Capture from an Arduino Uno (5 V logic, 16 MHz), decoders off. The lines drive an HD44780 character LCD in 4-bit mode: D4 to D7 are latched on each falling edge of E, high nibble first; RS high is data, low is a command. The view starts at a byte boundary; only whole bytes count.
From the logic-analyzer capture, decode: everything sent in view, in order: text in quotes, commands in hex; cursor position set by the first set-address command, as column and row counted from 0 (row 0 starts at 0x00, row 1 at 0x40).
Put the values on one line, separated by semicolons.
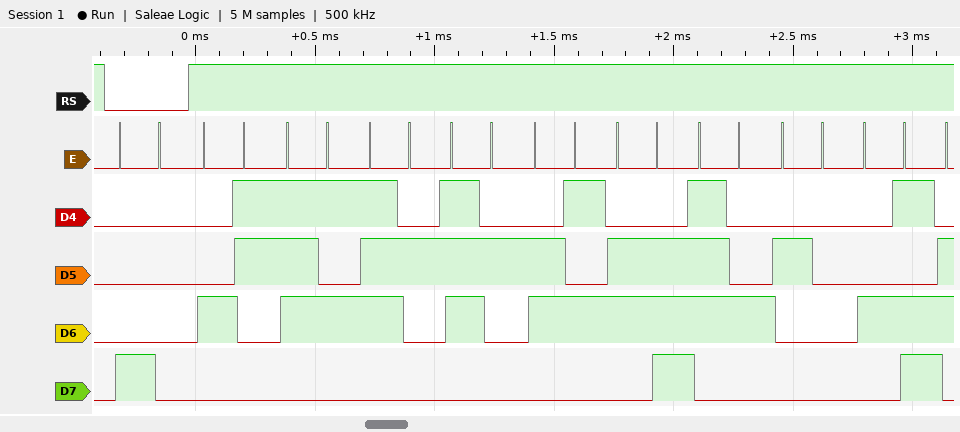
0x80 "Current M"; column 0, row 0
